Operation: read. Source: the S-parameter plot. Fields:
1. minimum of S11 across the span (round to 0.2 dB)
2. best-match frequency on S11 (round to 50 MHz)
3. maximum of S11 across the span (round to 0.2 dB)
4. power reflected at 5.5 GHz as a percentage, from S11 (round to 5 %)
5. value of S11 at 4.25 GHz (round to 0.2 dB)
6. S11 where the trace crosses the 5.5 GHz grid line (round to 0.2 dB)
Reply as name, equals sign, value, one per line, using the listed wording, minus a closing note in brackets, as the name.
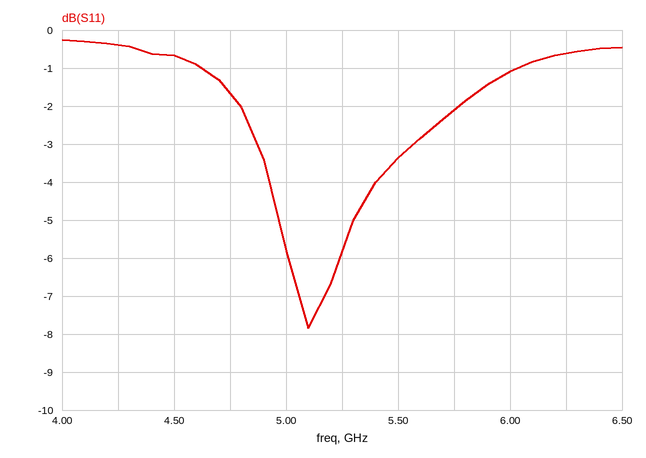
minimum of S11 across the span = -7.8 dB
best-match frequency on S11 = 5.10 GHz
maximum of S11 across the span = -0.2 dB
power reflected at 5.5 GHz as a percentage, from S11 = 45 %
value of S11 at 4.25 GHz = -0.4 dB
S11 where the trace crosses the 5.5 GHz grid line = -3.4 dB
